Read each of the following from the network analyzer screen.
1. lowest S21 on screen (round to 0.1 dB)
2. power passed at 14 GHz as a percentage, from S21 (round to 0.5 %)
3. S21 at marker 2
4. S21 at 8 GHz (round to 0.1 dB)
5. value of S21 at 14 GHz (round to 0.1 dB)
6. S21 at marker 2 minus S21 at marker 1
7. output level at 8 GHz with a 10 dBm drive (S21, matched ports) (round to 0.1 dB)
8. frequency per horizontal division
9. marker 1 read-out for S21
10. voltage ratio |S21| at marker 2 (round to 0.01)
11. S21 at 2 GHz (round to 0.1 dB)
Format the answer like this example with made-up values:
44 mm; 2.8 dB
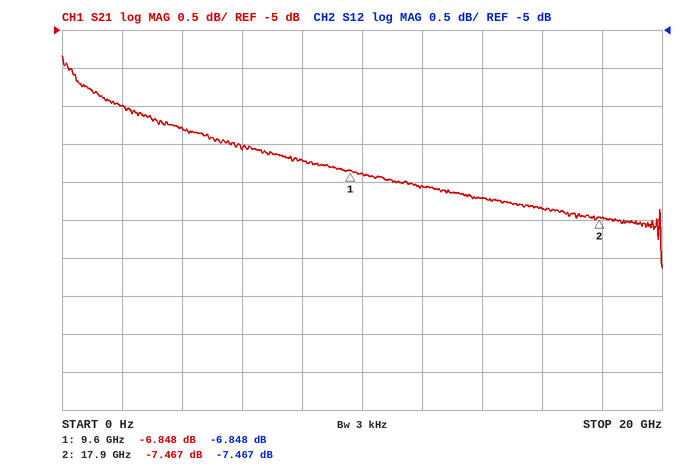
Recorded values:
-8.1 dB; 19.0 %; -7.467 dB; -6.7 dB; -7.2 dB; -0.619 dB; 3.3 dBm; 2 GHz; -6.848 dB; 0.42; -6.0 dB
